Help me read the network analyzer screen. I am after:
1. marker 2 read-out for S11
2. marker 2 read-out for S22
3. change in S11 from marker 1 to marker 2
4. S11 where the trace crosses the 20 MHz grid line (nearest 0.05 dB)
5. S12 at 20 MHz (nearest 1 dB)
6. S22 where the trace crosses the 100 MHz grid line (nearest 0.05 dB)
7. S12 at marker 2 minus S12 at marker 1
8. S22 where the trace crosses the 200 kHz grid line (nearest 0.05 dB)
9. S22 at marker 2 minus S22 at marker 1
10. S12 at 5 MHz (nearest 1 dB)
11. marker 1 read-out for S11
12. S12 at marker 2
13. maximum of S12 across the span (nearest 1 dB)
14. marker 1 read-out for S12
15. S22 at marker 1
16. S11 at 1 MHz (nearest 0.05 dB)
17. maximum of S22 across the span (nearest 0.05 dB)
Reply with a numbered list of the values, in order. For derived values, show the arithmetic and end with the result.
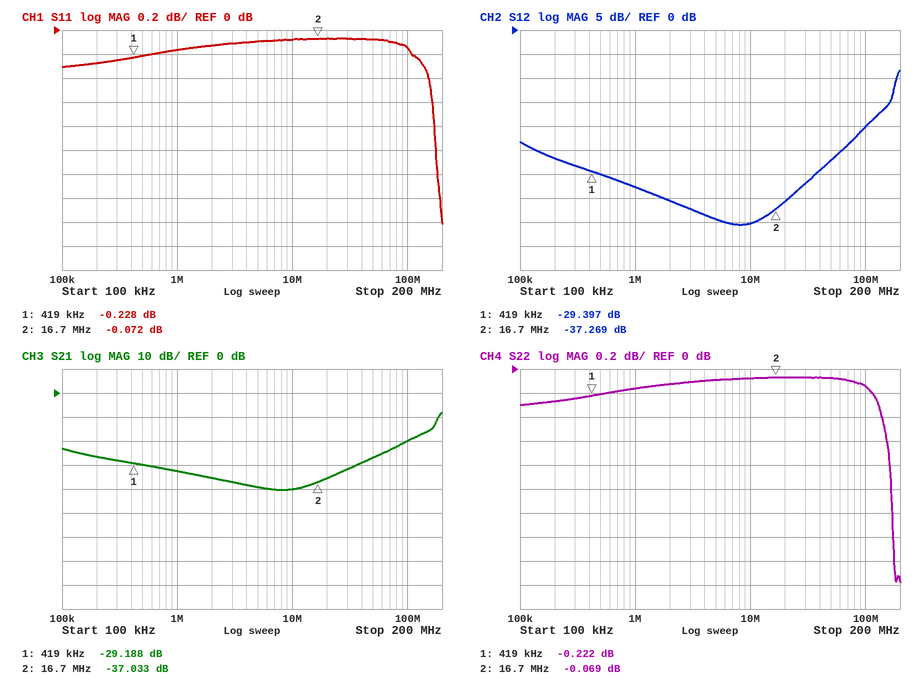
1. -0.072 dB
2. -0.069 dB
3. -0.072 − (-0.228) = 0.156 dB
4. -0.05 dB
5. -36 dB
6. -0.15 dB
7. -37.269 − (-29.397) = -7.872 dB
8. -0.25 dB
9. -0.069 − (-0.222) = 0.153 dB
10. -39 dB
11. -0.228 dB
12. -37.269 dB
13. -8 dB
14. -29.397 dB
15. -0.222 dB
16. -0.15 dB
17. -0.05 dB
